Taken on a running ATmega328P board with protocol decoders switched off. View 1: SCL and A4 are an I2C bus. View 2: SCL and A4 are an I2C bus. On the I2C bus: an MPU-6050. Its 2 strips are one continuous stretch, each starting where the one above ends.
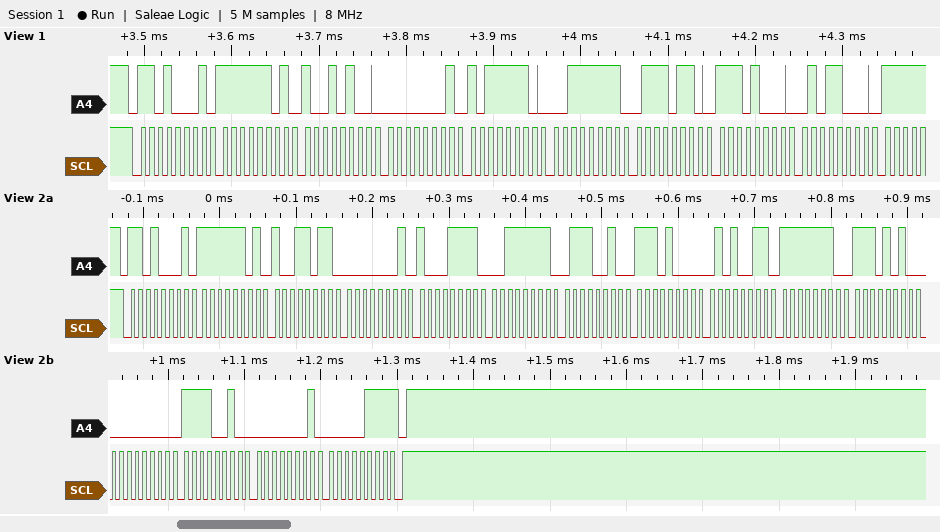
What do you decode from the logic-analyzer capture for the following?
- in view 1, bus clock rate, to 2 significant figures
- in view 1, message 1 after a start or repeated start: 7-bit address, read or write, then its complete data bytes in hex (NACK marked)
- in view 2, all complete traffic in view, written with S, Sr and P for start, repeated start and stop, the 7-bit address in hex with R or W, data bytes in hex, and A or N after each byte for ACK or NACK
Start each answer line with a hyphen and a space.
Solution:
- 100 kHz
- 0x68 read: FD 94 01 BE 3F 76 E8 58
- S 68R A FD A 9B A 01 A 8F A 3F A 72 A E8 A 53 A FE A EA A 00 A F2 A 01 A 07 N P
